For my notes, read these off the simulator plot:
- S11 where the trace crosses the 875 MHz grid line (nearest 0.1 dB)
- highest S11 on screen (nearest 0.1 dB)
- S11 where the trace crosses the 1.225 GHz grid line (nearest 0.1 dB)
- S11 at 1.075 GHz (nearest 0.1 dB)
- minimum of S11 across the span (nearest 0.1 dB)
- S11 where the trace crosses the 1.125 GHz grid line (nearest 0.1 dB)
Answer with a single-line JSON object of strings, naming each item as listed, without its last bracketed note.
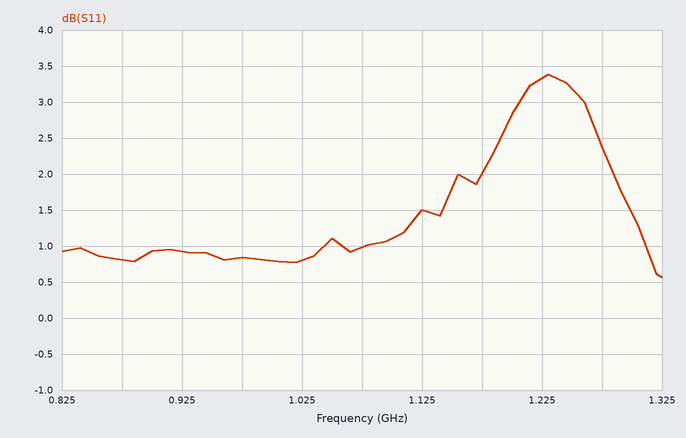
{"S11 where the trace crosses the 875 MHz grid line": "0.8 dB", "highest S11 on screen": "3.4 dB", "S11 where the trace crosses the 1.225 GHz grid line": "3.3 dB", "S11 at 1.075 GHz": "1.0 dB", "minimum of S11 across the span": "0.6 dB", "S11 where the trace crosses the 1.125 GHz grid line": "1.5 dB"}
